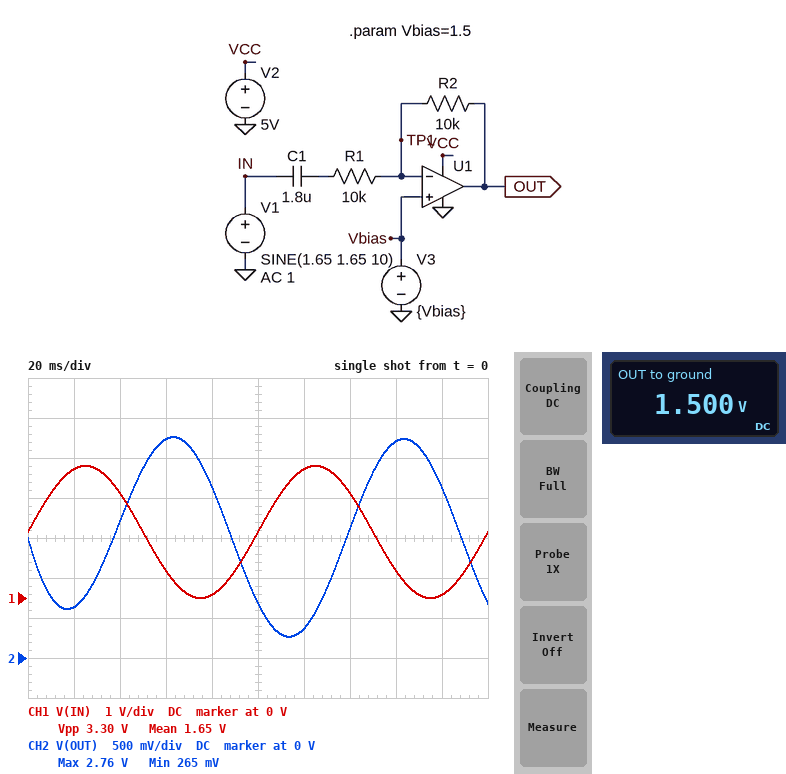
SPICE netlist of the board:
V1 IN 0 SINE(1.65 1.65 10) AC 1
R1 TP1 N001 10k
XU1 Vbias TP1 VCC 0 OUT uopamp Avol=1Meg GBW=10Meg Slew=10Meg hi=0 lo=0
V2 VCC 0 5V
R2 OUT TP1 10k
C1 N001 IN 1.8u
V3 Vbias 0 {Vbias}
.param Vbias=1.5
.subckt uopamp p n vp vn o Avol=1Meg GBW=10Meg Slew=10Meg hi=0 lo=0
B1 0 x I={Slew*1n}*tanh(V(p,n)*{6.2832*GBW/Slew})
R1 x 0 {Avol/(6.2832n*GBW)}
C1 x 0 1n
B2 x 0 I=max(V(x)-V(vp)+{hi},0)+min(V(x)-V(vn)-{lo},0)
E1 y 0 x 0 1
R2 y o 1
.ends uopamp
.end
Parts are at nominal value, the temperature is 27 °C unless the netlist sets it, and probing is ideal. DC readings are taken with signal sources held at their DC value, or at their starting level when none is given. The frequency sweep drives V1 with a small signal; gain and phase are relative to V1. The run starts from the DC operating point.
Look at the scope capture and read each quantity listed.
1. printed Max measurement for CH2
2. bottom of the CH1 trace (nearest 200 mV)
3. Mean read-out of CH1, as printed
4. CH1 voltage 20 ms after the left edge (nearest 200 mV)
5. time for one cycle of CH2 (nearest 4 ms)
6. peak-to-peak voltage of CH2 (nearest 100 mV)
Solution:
2.76 V
0 V
1.65 V
3.2 V
100 ms
2.5 V
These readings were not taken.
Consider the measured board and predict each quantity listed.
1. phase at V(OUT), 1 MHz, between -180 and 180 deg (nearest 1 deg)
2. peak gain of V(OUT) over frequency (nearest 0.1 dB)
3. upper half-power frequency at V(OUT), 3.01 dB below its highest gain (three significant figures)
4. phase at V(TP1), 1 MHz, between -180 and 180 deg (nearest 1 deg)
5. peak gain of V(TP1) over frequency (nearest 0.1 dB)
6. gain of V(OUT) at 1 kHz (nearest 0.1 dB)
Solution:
169 deg
0 dB
5.00 MHz
79 deg
-6.0 dB
0 dB
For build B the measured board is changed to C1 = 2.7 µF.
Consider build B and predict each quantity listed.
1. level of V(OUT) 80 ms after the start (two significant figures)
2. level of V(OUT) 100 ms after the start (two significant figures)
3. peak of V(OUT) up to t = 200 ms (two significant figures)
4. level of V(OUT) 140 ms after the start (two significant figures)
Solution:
2.5 V
800 mV
3.0 V
1.4 V
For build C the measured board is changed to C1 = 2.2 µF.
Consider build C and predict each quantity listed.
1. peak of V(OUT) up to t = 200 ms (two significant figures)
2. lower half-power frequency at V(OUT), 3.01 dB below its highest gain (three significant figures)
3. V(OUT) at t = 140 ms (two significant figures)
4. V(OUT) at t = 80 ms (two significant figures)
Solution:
2.9 V
7.23 Hz
1.5 V
2.3 V
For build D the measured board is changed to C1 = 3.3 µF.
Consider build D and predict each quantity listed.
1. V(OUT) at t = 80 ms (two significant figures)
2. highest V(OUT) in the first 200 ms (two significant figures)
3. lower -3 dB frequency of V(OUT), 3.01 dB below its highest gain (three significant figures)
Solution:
2.6 V
3.1 V
4.82 Hz
